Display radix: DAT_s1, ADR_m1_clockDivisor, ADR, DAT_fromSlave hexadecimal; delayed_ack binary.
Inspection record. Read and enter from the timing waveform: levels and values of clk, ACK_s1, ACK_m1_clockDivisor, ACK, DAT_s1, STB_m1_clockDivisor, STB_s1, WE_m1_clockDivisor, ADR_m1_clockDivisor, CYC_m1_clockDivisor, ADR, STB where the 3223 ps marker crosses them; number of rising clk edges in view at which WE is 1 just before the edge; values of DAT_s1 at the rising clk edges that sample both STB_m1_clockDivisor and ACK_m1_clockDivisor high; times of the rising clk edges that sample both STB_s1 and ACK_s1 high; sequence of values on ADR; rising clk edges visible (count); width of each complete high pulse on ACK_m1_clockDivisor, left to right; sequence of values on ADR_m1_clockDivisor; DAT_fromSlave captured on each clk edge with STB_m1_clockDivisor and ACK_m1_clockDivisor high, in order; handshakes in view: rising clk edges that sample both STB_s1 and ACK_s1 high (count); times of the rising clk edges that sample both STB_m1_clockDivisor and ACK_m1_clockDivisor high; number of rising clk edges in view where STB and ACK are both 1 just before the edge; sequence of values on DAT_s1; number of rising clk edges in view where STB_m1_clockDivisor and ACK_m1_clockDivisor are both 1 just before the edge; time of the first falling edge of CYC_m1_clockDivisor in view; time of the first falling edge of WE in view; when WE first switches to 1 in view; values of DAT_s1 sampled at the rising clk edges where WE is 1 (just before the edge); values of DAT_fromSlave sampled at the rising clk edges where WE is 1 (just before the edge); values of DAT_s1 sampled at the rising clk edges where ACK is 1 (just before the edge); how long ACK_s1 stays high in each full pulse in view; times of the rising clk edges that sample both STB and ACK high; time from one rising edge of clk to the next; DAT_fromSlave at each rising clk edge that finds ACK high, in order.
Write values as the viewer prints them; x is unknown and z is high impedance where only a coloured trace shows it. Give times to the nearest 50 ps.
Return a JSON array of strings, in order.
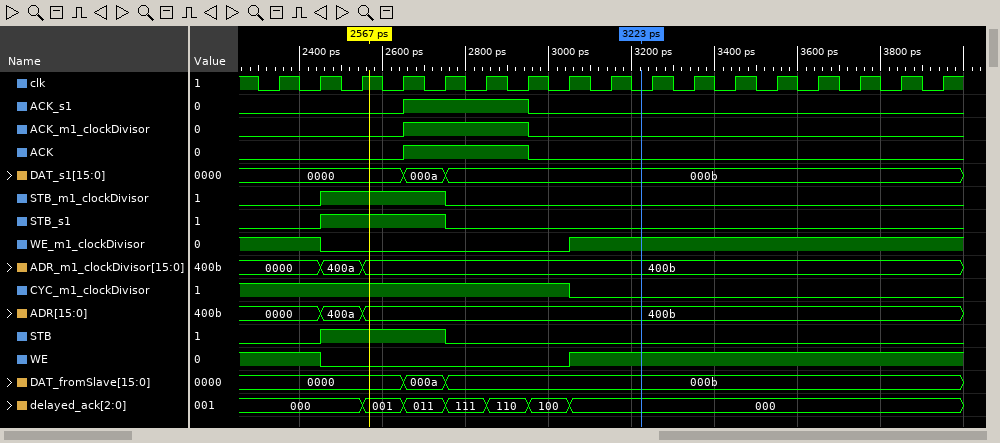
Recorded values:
["clk=0, ACK_s1=0, ACK_m1_clockDivisor=0, ACK=0, DAT_s1=000b, STB_m1_clockDivisor=0, STB_s1=0, WE_m1_clockDivisor=1, ADR_m1_clockDivisor=400b, CYC_m1_clockDivisor=0, ADR=400b, STB=0", "11", "000a", "2750 ps", "0000, 400a, 400b", "17", "300 ps", "0000, 400a, 400b", "000a", "1", "2750 ps", "1", "0000, 000a, 000b", "1", "3050 ps", "2450 ps", "3050 ps", "0000, 0000, 000b, 000b, 000b, 000b, 000b, 000b, 000b, 000b, 000b", "0000, 0000, 000b, 000b, 000b, 000b, 000b, 000b, 000b, 000b, 000b", "000a, 000b, 000b", "300 ps", "2750 ps", "100 ps", "000a, 000b, 000b"]
